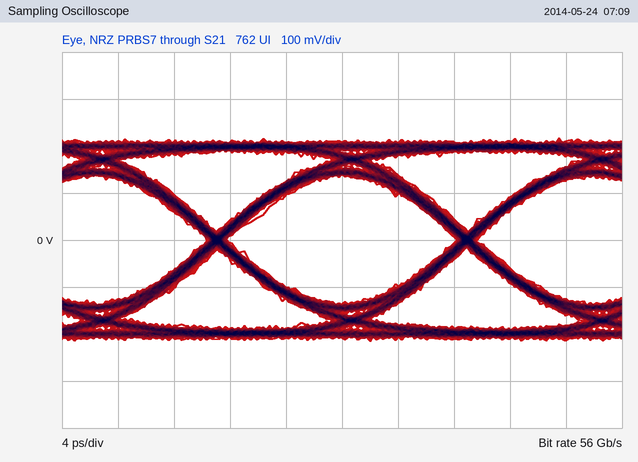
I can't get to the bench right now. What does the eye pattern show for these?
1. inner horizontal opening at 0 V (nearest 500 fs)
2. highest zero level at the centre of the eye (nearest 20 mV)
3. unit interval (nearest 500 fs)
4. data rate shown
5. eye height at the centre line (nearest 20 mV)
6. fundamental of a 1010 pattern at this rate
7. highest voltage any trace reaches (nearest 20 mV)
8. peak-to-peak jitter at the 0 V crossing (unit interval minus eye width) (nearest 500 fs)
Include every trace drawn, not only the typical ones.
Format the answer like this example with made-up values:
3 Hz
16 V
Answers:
16.5 ps
-140 mV
18.0 ps
56 Gb/s
280 mV
28 GHz
220 mV
1.5 ps
